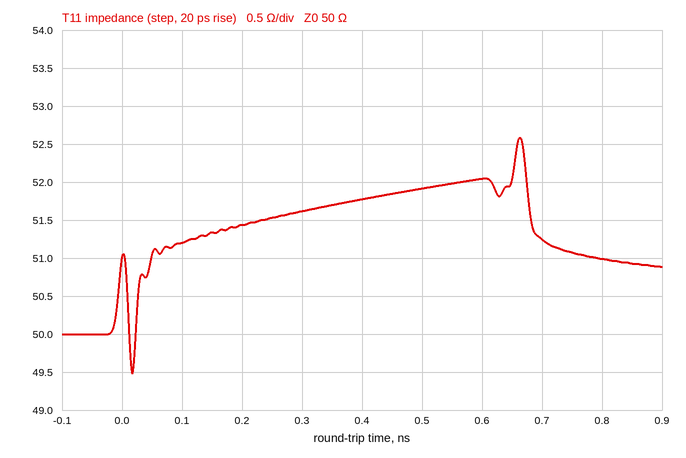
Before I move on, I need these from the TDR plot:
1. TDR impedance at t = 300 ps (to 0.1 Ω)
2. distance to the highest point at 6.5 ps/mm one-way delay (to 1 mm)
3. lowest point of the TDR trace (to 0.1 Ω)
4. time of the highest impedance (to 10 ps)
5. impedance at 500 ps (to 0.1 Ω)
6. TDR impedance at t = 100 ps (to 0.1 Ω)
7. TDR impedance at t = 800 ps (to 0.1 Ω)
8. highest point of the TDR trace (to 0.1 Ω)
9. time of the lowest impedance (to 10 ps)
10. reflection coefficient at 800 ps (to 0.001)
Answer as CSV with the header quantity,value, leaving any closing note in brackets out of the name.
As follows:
quantity,value
TDR impedance at t = 300 ps,51.6 Ω
distance to the highest point at 6.5 ps/mm one-way delay,51 mm
lowest point of the TDR trace,49.5 Ω
time of the highest impedance,660 ps
impedance at 500 ps,51.9 Ω
TDR impedance at t = 100 ps,51.2 Ω
TDR impedance at t = 800 ps,51.0 Ω
highest point of the TDR trace,52.6 Ω
time of the lowest impedance,20 ps
reflection coefficient at 800 ps,+0.010
